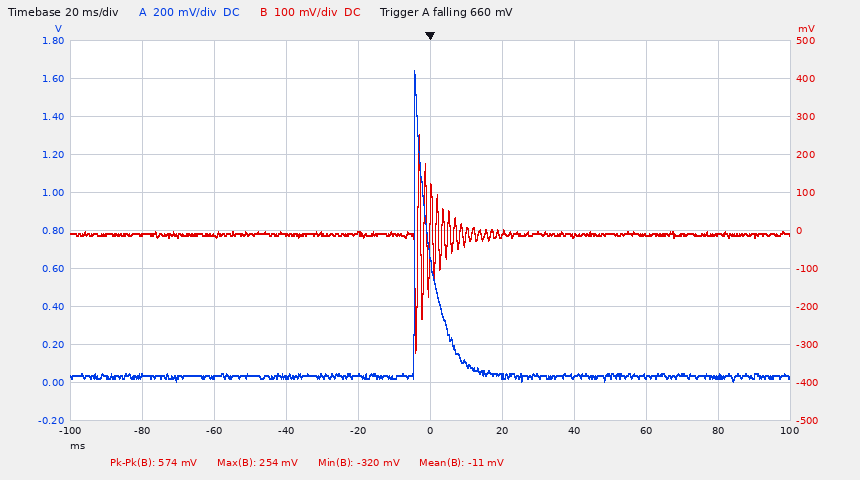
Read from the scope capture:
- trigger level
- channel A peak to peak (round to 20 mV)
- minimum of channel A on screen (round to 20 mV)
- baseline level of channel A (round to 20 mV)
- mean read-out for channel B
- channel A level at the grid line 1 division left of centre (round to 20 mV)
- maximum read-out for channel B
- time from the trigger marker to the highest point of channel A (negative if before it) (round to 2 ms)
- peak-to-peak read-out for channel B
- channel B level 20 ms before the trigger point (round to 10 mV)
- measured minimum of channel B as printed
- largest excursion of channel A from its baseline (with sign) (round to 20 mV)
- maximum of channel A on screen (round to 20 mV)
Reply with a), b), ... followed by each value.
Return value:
a) 660 mV
b) 1.64 V
c) 0 mV
d) 40 mV
e) -11 mV
f) 40 mV
g) 254 mV
h) -4 ms
i) 574 mV
j) -10 mV
k) -320 mV
l) +1.60 V
m) 1.64 V
